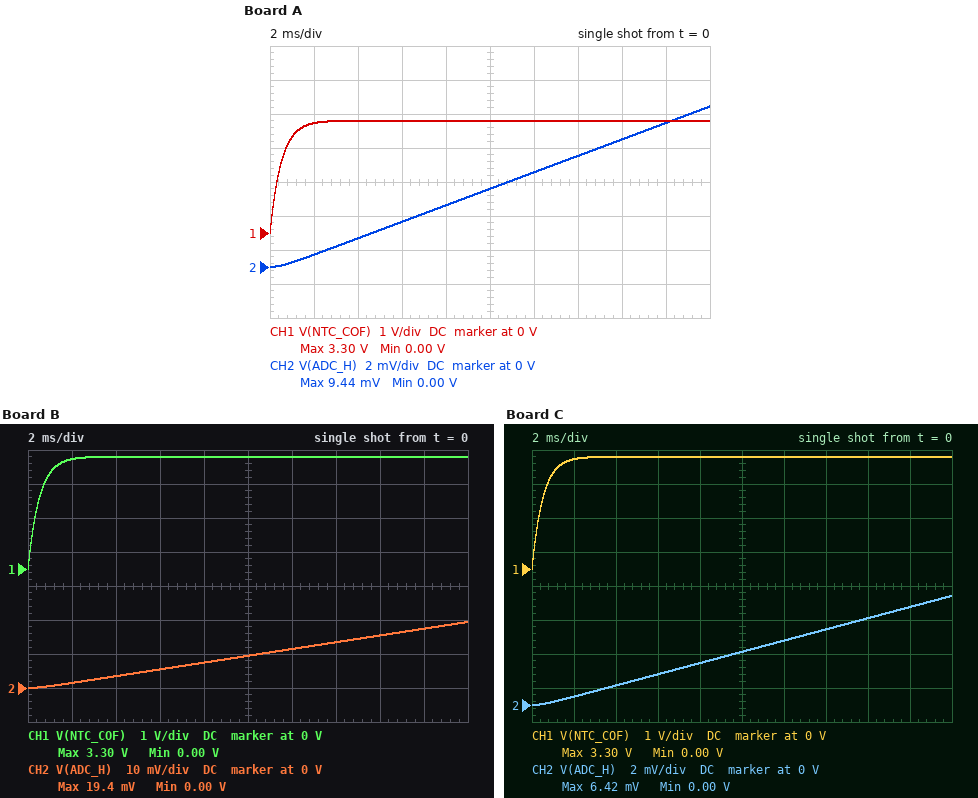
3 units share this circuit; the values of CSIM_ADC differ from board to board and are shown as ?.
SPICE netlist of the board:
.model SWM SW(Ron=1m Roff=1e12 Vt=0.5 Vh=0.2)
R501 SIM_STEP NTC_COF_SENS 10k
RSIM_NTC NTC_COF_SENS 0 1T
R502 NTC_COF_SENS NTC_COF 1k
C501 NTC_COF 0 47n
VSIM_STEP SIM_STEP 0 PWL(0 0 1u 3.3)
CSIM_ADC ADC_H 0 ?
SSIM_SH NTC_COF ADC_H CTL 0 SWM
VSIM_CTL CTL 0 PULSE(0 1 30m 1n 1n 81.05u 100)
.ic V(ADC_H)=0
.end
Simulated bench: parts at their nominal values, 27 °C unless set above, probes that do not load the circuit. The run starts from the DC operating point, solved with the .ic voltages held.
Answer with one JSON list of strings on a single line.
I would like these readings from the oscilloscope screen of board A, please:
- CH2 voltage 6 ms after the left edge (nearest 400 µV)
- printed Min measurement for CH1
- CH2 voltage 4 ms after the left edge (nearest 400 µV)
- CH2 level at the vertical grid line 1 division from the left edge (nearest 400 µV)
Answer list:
["2.8 mV", "0.00 V", "1.6 mV", "800 µV"]
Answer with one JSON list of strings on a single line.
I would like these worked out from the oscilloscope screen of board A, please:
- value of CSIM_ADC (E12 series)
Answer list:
["6.8 pF"]
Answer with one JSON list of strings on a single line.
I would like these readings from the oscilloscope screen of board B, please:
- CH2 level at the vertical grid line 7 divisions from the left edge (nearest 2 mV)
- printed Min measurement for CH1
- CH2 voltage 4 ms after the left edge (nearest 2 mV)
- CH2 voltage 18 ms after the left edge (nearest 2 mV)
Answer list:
["14 mV", "0.00 V", "4 mV", "18 mV"]
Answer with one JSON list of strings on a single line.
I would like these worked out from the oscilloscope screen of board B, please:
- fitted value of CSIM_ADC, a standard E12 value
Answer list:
["3.3 pF"]
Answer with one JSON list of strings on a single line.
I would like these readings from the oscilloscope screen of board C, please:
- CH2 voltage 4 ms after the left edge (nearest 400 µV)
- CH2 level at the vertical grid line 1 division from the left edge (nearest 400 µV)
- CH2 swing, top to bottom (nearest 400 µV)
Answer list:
["1.2 mV", "400 µV", "6.4 mV"]
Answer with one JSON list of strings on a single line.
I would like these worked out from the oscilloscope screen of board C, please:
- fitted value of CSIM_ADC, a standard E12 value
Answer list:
["10 pF"]
